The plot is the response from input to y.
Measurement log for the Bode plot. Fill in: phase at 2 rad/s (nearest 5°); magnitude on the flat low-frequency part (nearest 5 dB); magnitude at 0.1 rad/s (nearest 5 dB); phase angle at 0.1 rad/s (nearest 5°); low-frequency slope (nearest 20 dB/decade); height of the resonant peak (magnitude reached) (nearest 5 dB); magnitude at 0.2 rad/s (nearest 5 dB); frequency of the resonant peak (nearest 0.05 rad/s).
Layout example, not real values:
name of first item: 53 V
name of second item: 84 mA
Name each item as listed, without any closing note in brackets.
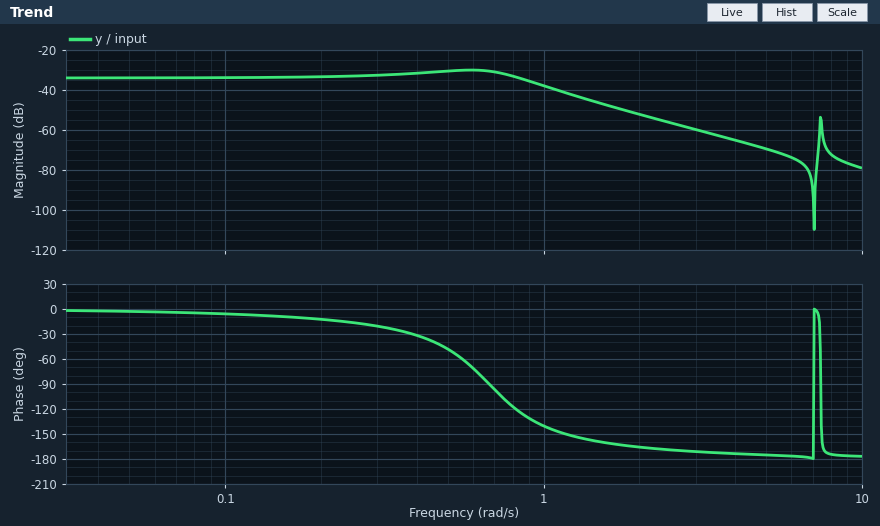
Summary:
phase at 2 rad/s: -165°
magnitude on the flat low-frequency part: -35 dB
magnitude at 0.1 rad/s: -35 dB
phase angle at 0.1 rad/s: -5°
low-frequency slope: 0 dB/decade
height of the resonant peak (magnitude reached): -30 dB
magnitude at 0.2 rad/s: -35 dB
frequency of the resonant peak: 0.60 rad/s
